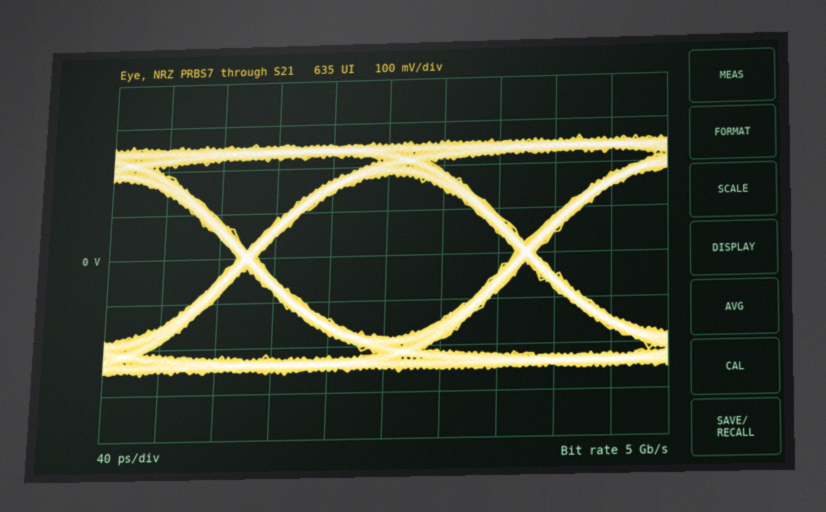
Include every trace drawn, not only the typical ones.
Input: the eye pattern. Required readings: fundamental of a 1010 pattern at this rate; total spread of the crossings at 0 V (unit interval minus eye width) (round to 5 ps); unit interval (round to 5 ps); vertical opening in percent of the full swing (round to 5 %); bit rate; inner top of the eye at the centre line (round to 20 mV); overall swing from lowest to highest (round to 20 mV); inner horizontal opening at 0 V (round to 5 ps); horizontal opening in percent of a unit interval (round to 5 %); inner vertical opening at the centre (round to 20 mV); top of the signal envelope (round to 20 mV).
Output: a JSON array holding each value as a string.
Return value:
["2.5 GHz", "15 ps", "200 ps", "70 %", "5 Gb/s", "180 mV", "520 mV", "185 ps", "90 %", "360 mV", "260 mV"]
